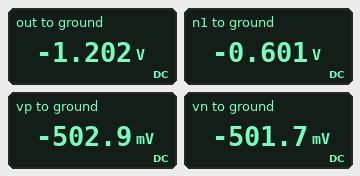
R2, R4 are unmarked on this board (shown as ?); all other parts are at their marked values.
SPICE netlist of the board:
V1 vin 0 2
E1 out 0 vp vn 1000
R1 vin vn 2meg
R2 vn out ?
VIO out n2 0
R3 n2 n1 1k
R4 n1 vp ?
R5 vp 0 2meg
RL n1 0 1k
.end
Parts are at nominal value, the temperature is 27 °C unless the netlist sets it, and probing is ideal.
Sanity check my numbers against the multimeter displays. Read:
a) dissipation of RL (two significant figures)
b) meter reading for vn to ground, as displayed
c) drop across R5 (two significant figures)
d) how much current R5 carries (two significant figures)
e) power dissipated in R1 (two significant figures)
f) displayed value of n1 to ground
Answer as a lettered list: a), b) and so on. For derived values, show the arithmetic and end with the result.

a) (0 V - (-601 mV))^2 / 1 kΩ = 360 µW
b) -501.7 mV
c) 0 V - (-502.9 mV) = 500 mV
d) (0 V - (-502.9 mV)) / 2 MΩ = 250 nA
e) (2 V - (-501.7 mV))^2 / 2 MΩ = 3.1 µW
f) -0.601 V
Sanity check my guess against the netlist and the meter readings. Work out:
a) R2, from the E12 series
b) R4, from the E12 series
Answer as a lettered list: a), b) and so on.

a) 560 kΩ
b) 390 kΩ
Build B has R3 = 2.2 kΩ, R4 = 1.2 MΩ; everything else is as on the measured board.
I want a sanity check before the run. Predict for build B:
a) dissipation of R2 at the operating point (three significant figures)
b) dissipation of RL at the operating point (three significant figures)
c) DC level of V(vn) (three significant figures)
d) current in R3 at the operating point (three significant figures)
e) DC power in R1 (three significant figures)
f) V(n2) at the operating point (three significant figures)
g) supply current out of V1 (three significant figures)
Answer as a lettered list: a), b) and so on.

a) 644 nW
b) 54.2 µW
c) -145 mV
d) 233 µA
e) 2.30 µW
f) -745 mV
g) 1.07 µA
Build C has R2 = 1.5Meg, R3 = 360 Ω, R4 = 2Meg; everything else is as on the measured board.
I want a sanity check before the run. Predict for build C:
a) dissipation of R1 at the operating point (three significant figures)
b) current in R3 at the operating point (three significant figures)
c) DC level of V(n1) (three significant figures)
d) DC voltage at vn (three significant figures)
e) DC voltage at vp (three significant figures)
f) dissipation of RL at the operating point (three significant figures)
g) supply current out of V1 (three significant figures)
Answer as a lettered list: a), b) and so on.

a) 6.25 µW
b) 3.08 mA
c) -3.08 V
d) -1.53 V
e) -1.54 V
f) 9.47 mW
g) 1.77 µA
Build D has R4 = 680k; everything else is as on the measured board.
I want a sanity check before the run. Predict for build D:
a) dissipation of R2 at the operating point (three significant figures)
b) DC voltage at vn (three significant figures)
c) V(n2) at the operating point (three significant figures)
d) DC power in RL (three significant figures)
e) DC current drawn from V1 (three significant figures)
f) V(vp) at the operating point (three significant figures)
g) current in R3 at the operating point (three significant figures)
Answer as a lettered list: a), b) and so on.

a) 805 nW
b) -398 mV
c) -1.07 V
d) 286 µW
e) 1.20 µA
f) -399 mV
g) 535 µA
